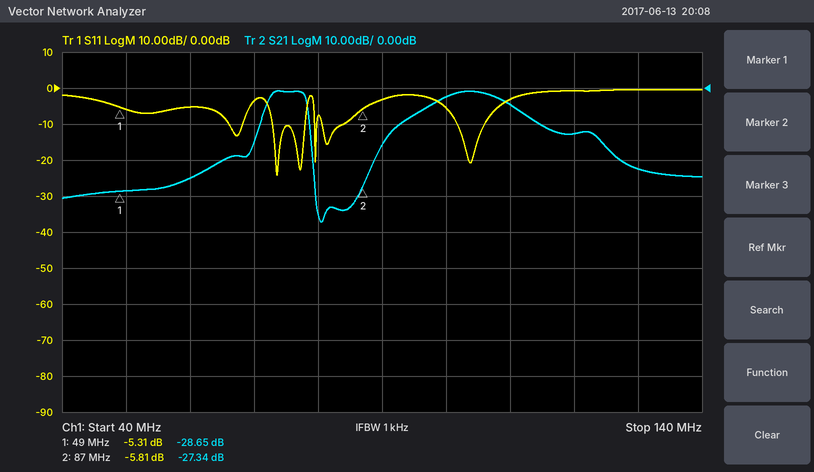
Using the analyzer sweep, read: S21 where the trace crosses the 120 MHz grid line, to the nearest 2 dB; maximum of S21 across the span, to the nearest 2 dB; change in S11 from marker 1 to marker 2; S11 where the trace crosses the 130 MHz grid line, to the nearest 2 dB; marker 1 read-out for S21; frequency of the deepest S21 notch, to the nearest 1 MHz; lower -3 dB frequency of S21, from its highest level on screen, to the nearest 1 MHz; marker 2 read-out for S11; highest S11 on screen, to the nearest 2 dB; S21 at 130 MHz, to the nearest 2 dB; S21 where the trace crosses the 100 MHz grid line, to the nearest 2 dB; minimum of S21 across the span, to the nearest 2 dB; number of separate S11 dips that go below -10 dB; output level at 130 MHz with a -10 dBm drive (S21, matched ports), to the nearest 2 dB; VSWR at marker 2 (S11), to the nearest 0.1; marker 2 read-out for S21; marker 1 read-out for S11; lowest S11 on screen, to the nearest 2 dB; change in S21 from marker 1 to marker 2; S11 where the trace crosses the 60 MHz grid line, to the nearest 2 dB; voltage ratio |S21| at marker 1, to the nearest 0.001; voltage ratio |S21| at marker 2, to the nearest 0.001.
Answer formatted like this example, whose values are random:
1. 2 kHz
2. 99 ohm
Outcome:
1. -12 dB
2. 0 dB
3. -0.50 dB
4. 0 dB
5. -28.65 dB
6. 81 MHz
7. 72 MHz
8. -5.81 dB
9. 0 dB
10. -22 dB
11. -2 dB
12. -38 dB
13. 6
14. -32 dBm
15. 3.1
16. -27.34 dB
17. -5.31 dB
18. -24 dB
19. 1.31 dB
20. -6 dB
21. 0.037
22. 0.043
